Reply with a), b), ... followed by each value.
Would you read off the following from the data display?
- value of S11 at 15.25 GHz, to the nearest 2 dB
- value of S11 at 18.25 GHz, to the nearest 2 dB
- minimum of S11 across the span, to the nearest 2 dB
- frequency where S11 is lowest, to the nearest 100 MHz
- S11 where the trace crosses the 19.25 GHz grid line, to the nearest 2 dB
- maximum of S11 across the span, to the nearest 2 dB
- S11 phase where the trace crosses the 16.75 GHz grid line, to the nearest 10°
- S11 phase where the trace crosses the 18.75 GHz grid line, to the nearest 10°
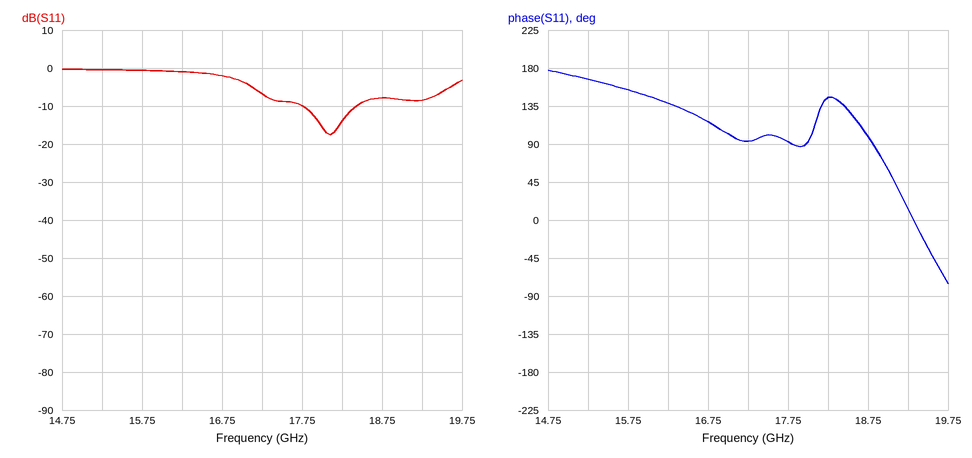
a) 0 dB
b) -14 dB
c) -18 dB
d) 18.1 GHz
e) -8 dB
f) 0 dB
g) 120°
h) 100°
